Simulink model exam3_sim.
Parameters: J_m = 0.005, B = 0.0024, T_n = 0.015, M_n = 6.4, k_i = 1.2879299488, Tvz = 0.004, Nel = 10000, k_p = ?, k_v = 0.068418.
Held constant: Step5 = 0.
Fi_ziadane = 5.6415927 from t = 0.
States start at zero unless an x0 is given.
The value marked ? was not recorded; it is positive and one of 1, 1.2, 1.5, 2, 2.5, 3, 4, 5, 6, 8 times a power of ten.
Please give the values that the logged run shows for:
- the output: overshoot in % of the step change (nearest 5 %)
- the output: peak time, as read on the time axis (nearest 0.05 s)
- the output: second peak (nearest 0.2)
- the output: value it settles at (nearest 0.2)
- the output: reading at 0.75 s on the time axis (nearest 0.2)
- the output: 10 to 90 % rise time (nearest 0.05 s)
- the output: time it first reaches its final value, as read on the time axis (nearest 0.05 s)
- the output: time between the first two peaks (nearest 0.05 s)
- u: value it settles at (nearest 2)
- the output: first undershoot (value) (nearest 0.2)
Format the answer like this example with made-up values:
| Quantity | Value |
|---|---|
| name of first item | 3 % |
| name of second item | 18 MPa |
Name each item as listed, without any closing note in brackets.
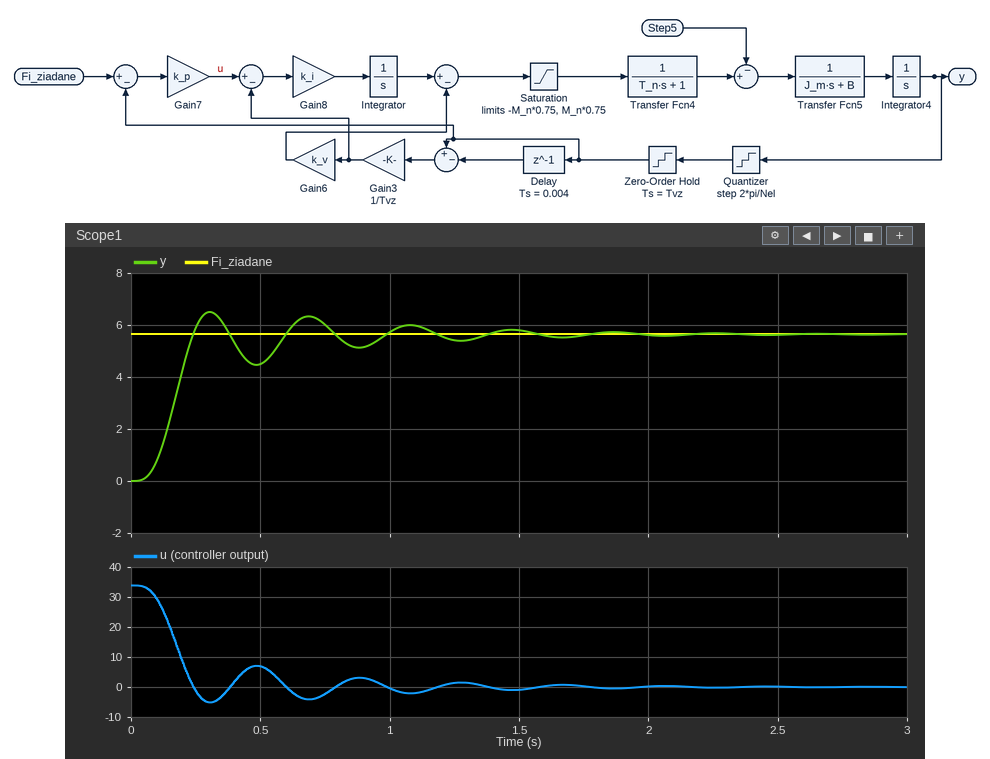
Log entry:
| Quantity | Value |
|---|---|
| the output: overshoot in % of the step change | 15 % |
| the output: peak time, as read on the time axis | 0.30 s |
| the output: second peak | 6.4 |
| the output: value it settles at | 5.6 |
| the output: reading at 0.75 s on the time axis | 6.0 |
| the output: 10 to 90 % rise time | 0.15 s |
| the output: time it first reaches its final value, as read on the time axis | 0.25 s |
| the output: time between the first two peaks | 0.40 s |
| u: value it settles at | 0 |
| the output: first undershoot (value) | 4.4 |
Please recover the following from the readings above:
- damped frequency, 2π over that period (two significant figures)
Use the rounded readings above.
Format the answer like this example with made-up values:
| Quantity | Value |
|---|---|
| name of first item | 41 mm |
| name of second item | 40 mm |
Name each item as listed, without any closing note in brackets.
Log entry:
| Quantity | Value |
|---|---|
| damped frequency, 2π over that period | 16 rad/s |
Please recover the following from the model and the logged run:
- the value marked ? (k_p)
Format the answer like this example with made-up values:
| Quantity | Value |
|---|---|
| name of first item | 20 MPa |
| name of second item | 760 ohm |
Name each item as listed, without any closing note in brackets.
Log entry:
| Quantity | Value |
|---|---|
| the value marked ? | 6 |
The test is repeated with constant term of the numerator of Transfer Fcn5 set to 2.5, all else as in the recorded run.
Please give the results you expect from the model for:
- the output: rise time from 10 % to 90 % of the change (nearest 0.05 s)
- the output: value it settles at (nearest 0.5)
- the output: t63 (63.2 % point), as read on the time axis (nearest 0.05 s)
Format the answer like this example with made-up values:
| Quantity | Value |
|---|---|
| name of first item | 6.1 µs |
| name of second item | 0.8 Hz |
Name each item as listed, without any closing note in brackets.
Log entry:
| Quantity | Value |
|---|---|
| the output: rise time from 10 % to 90 % of the change | 0.25 s |
| the output: value it settles at | 5.5 |
| the output: t63 (63.2 % point), as read on the time axis | 0.15 s |
